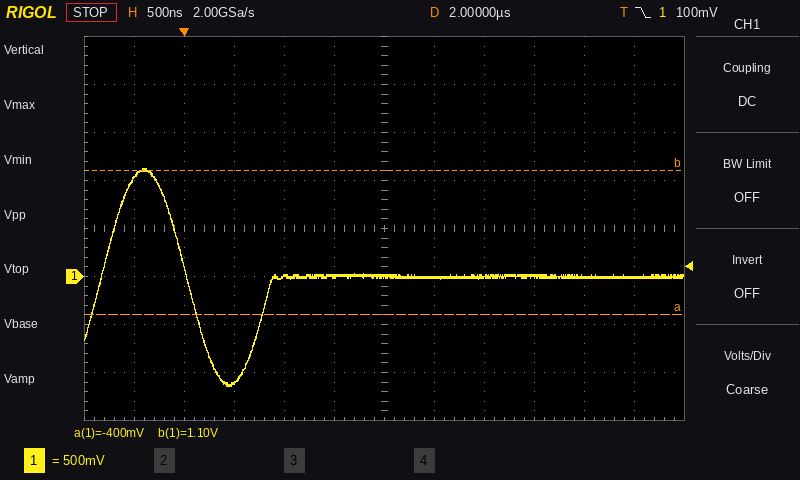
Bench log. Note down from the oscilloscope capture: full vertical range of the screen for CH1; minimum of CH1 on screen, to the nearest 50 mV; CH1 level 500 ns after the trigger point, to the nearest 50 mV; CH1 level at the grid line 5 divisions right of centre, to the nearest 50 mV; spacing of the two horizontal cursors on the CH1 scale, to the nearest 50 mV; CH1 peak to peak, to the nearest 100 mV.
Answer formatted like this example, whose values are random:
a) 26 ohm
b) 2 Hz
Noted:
a) 4 V
b) -1.15 V
c) -1.10 V
d) 0 mV
e) 1.50 V
f) 2.30 V
